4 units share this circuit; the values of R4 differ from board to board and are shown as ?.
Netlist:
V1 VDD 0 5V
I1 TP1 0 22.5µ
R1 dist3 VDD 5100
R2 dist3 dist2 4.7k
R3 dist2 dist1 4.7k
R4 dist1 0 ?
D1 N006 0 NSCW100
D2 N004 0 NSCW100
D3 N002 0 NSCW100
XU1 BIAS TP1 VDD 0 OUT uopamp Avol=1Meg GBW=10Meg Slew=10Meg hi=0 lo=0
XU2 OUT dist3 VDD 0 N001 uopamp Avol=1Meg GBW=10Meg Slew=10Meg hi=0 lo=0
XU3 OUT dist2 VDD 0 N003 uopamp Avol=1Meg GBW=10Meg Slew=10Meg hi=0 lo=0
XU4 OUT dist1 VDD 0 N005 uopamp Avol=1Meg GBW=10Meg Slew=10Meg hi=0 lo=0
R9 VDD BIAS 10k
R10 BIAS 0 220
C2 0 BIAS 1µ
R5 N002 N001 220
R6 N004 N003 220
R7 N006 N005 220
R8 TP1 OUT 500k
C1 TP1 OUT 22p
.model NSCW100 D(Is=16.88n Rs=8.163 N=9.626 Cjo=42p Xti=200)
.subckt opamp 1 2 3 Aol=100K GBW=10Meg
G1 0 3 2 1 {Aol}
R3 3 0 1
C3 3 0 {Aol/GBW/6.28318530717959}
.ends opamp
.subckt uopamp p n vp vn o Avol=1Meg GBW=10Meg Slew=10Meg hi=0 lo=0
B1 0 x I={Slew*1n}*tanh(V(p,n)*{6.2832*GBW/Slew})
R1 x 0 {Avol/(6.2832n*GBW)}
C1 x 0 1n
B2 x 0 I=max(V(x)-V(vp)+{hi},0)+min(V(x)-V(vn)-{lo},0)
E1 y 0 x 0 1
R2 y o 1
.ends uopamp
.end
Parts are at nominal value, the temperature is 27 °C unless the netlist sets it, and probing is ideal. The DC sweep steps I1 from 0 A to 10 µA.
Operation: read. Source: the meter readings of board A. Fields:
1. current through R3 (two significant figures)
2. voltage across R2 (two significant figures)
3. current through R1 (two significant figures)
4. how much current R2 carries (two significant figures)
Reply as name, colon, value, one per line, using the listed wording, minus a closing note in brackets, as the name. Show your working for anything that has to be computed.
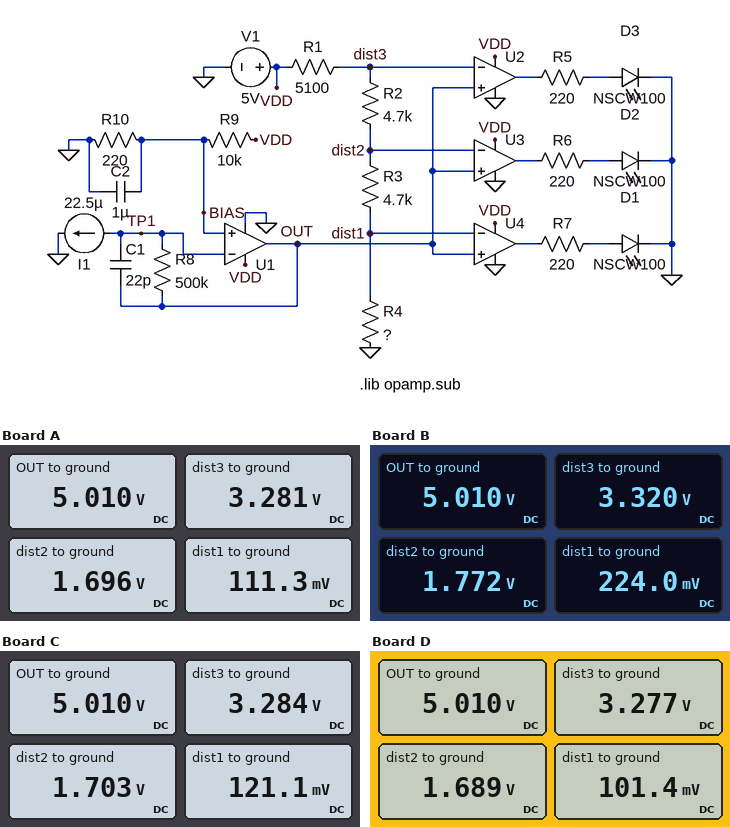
current through R3: (1.696 V - 111.3 mV) / 4.7 kΩ = 340 µA
voltage across R2: 3.281 V - 1.696 V = 1.6 V
current through R1: (5 V - 3.281 V) / 5.1 kΩ = 340 µA
how much current R2 carries: (3.281 V - 1.696 V) / 4.7 kΩ = 340 µA
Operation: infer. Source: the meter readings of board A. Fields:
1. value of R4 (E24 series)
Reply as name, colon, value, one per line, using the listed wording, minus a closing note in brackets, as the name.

value of R4: 330 Ω
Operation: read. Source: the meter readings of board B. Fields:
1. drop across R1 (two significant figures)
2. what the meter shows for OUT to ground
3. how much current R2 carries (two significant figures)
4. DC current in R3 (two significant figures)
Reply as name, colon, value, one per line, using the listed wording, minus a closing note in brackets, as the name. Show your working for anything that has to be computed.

drop across R1: 5 V - 3.32 V = 1.7 V
what the meter shows for OUT to ground: 5.010 V
how much current R2 carries: (3.32 V - 1.772 V) / 4.7 kΩ = 330 µA
DC current in R3: (1.772 V - 224 mV) / 4.7 kΩ = 330 µA
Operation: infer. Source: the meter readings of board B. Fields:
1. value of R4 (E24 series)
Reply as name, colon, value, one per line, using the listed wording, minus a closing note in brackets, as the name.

value of R4: 680 Ω
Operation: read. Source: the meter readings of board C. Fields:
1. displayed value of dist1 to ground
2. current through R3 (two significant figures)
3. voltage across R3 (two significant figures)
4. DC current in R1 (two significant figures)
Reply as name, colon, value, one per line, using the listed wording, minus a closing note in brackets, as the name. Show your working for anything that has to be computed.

displayed value of dist1 to ground: 121.1 mV
current through R3: (1.703 V - 121.1 mV) / 4.7 kΩ = 340 µA
voltage across R3: 1.703 V - 121.1 mV = 1.6 V
DC current in R1: (5 V - 3.284 V) / 5.1 kΩ = 340 µA
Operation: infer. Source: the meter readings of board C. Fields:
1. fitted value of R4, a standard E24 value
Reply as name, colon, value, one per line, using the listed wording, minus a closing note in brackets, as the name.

fitted value of R4, a standard E24 value: 360 Ω
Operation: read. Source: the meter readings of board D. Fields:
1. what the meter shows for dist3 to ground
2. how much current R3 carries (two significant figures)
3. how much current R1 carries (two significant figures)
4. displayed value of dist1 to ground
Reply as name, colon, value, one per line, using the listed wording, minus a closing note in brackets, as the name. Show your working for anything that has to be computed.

what the meter shows for dist3 to ground: 3.277 V
how much current R3 carries: (1.689 V - 101.4 mV) / 4.7 kΩ = 340 µA
how much current R1 carries: (5 V - 3.277 V) / 5.1 kΩ = 340 µA
displayed value of dist1 to ground: 101.4 mV
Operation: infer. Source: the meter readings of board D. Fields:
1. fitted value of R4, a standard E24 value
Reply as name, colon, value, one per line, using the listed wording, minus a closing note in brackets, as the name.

fitted value of R4, a standard E24 value: 300 Ω
